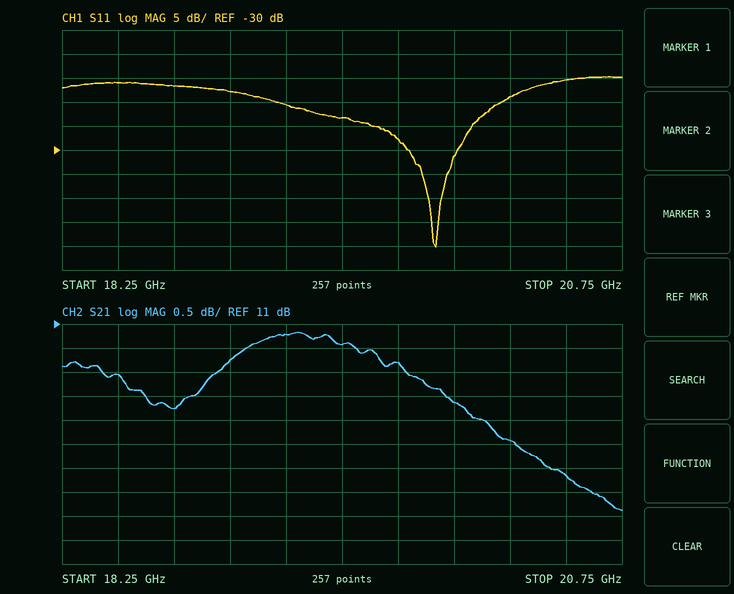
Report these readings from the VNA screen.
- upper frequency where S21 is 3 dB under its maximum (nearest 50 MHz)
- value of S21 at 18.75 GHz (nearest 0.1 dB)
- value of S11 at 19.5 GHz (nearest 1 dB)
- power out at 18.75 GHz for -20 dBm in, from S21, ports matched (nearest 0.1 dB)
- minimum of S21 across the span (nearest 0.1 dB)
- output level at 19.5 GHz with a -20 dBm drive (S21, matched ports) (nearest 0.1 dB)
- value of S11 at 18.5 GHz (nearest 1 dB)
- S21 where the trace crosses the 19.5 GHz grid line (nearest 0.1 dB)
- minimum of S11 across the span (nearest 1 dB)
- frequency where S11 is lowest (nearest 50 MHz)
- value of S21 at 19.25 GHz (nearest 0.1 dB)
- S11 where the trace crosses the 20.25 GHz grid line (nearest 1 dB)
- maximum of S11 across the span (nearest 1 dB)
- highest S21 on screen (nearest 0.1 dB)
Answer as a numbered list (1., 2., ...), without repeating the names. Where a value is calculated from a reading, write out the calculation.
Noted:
1. 20.50 GHz
2. 9.2 dB
3. -23 dB
4. -20 dBm + (9.2 dB) = -10.8 dBm
5. 7.1 dB
6. -20 dBm + (10.6 dB) = -9.4 dBm
7. -16 dB
8. 10.6 dB
9. -50 dB
10. 19.90 GHz
11. 10.8 dB
12. -19 dB
13. -15 dB
14. 10.8 dB
